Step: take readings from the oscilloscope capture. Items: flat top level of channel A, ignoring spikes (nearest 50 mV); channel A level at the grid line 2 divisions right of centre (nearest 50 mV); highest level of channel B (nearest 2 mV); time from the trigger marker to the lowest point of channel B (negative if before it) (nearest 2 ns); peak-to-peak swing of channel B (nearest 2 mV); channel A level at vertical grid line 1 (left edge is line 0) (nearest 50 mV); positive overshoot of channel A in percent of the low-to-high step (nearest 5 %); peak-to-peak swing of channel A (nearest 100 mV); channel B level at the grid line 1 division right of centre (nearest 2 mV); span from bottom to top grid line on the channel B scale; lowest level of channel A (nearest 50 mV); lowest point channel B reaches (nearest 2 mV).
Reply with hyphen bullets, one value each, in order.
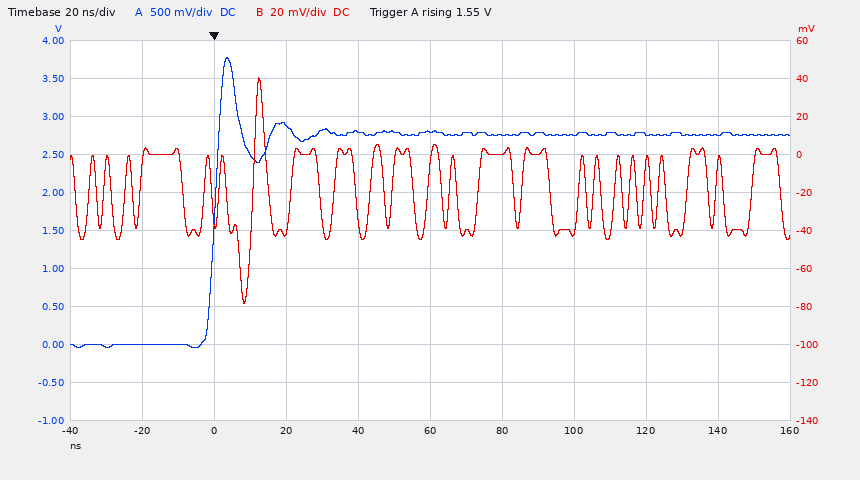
- 2.75 V
- 2.75 V
- 40 mV
- +8 ns
- 118 mV
- 0 mV
- 35 %
- 3.80 V
- 0 mV
- 200 mV
- -50 mV
- -78 mV
